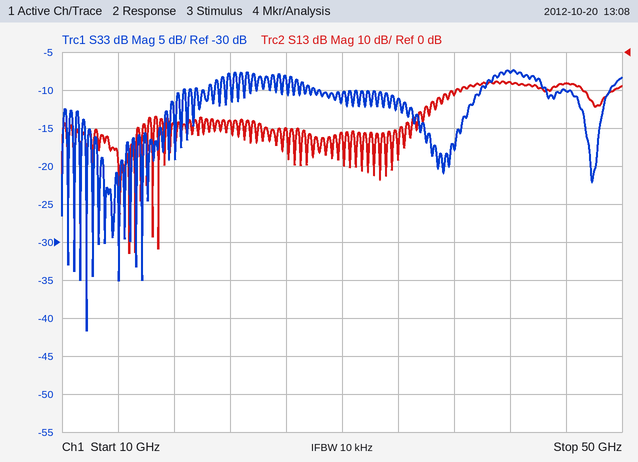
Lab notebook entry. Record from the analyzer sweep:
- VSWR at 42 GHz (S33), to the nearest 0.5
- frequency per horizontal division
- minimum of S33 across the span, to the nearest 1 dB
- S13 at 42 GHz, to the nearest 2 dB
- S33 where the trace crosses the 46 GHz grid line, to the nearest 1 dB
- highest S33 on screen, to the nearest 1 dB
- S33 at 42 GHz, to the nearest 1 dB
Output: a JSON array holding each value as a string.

["2.5", "4 GHz", "-42 dB", "-8 dB", "-10 dB", "-7 dB", "-8 dB"]
